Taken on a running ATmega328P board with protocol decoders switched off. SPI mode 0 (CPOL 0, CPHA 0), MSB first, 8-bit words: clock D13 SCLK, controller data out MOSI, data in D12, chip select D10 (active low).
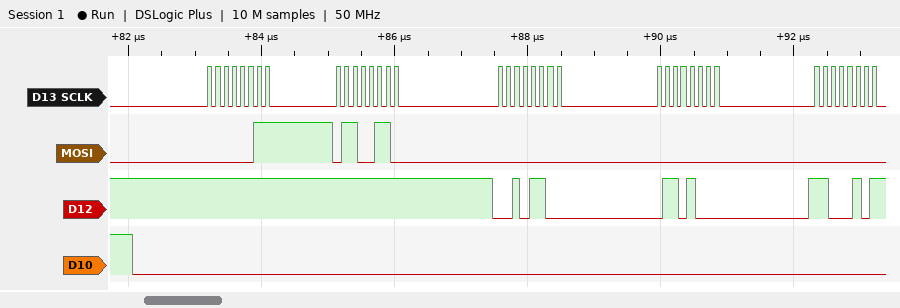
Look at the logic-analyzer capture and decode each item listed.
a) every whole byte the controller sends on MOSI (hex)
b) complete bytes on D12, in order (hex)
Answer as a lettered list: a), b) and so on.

a) 03 66 00 00 00
b) FF FF 2C 68 C5
